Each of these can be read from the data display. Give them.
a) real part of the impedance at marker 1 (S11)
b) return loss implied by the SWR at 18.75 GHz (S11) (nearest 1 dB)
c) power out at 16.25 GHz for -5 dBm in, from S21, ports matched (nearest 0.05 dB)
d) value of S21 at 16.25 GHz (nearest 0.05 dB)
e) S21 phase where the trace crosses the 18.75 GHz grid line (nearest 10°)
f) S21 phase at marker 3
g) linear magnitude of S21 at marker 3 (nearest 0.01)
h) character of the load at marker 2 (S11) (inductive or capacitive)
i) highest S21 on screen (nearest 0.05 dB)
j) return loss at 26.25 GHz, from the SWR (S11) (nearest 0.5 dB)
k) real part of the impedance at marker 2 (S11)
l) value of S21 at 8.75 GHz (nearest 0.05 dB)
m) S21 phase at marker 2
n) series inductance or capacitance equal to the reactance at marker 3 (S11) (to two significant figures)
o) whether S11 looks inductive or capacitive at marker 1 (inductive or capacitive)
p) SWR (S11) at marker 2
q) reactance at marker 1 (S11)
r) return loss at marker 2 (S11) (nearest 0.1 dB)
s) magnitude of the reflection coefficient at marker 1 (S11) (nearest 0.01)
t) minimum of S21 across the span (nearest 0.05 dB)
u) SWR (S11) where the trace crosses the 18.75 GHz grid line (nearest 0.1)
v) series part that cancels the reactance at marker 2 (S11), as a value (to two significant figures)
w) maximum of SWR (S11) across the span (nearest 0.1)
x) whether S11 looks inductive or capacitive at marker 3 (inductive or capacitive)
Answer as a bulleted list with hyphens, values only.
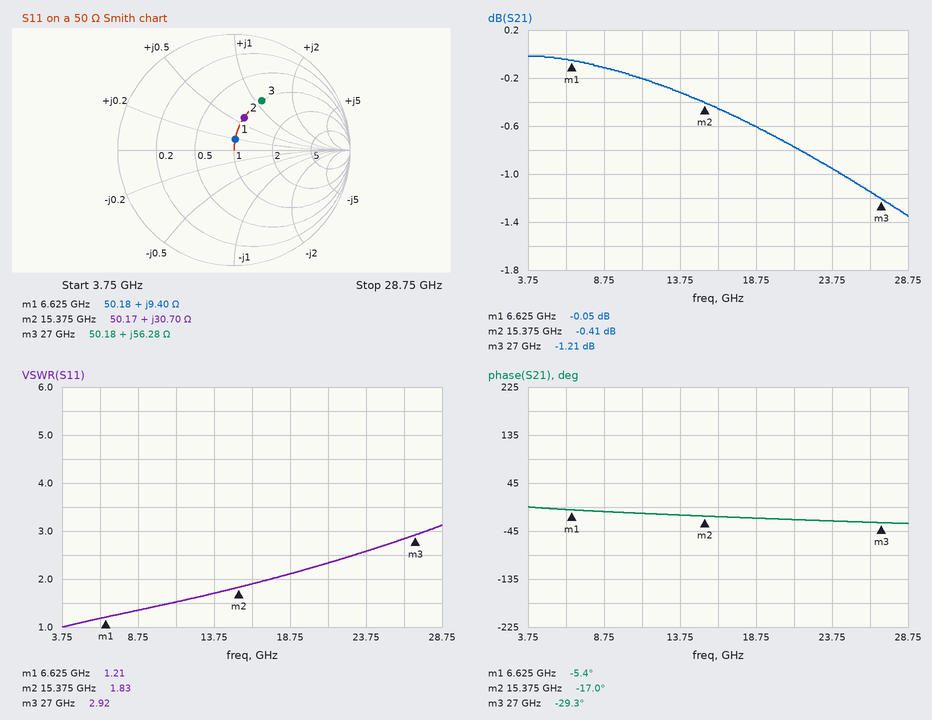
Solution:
- 50.18 Ω
- 9 dB
- -5.45 dBm
- -0.45 dB
- -20°
- -29.3°
- 0.87
- inductive
- 0.00 dB
- 6.5 dB
- 50.17 Ω
- -0.10 dB
- -17.0°
- 330 pH
- inductive
- 1.83
- +9.40 Ω
- 10.7 dB
- 0.09
- -1.35 dB
- 2.1
- 340 fF
- 3.1
- inductive
